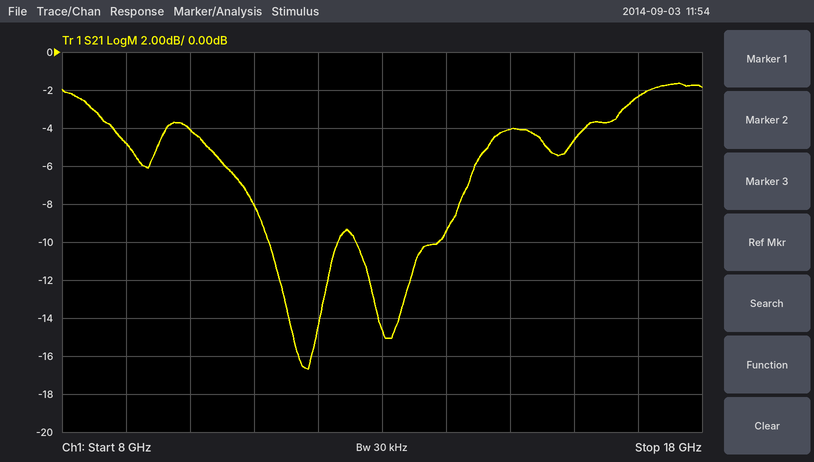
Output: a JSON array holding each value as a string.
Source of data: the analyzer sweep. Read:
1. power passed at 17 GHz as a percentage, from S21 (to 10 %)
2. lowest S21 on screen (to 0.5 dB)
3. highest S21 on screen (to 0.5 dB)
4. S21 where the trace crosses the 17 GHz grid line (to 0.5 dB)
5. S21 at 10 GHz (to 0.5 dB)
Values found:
["60 %", "-16.5 dB", "-1.5 dB", "-2.5 dB", "-4.0 dB"]
